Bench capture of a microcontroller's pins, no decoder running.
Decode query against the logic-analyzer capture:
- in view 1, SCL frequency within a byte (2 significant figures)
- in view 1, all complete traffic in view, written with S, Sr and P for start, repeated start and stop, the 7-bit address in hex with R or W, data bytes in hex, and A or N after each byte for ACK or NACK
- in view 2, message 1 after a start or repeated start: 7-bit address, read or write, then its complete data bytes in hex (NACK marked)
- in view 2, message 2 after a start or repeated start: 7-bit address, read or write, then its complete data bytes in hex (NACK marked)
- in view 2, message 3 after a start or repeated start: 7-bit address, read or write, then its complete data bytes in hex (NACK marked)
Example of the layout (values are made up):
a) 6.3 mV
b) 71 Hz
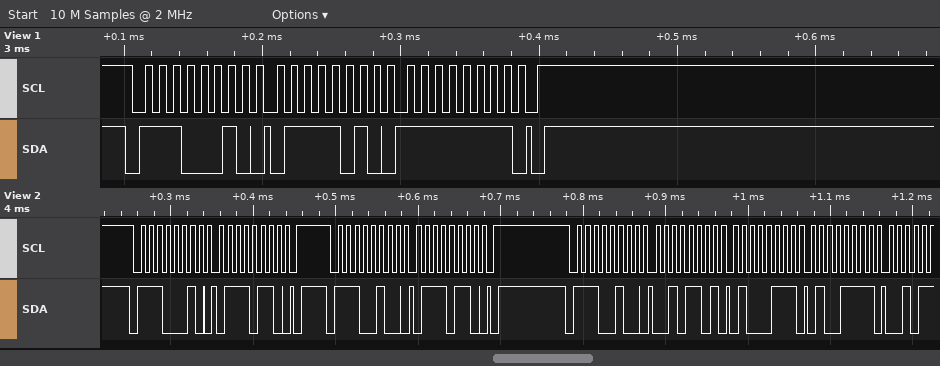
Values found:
a) 100 kHz
b) S 71W A 7A A FF A P
c) 0x71 write: 76
d) 0x72 write: 76
e) 0x72 write: 2D 47 4F
